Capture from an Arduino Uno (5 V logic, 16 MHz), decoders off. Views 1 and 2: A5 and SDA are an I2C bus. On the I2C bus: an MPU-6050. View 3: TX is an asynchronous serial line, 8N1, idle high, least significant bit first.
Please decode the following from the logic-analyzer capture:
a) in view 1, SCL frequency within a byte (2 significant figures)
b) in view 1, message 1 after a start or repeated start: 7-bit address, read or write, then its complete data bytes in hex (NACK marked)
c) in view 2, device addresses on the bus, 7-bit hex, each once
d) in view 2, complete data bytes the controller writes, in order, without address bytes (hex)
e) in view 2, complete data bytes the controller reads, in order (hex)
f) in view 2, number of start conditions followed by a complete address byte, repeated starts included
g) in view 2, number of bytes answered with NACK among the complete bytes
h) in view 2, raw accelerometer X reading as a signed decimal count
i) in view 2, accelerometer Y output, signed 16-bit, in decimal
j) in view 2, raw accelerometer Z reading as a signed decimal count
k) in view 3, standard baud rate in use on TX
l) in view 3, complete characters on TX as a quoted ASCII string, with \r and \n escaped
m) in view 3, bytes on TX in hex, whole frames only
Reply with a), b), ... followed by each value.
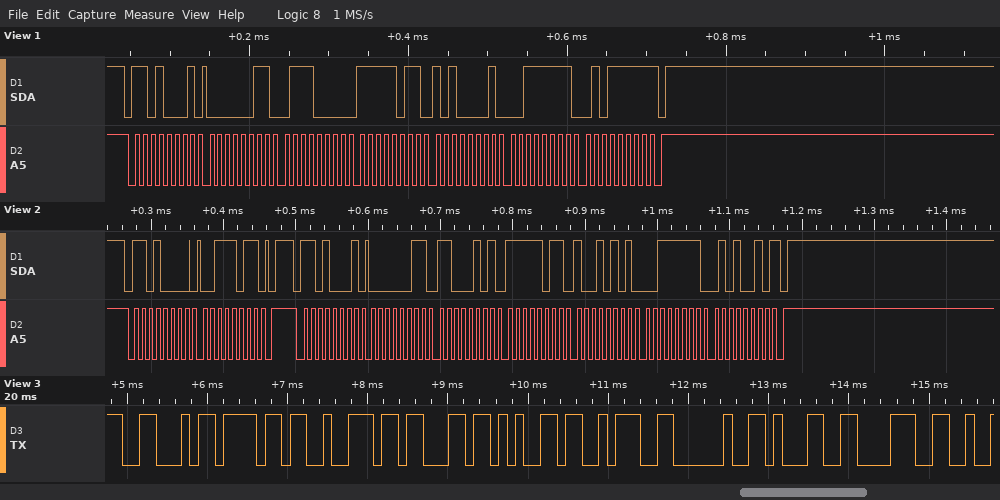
a) 100 kHz
b) 0x68 read: 03 70 FB A1 3F 5F NACK
c) 0x68
d) 3B
e) 03 C5 FB 95 3F 52
f) 2
g) 1
h) 965
i) -1131
j) 16210
k) 9600 baud
l) "Force: 18"
m) 46 6F 72 63 65 3A 20 31 38
